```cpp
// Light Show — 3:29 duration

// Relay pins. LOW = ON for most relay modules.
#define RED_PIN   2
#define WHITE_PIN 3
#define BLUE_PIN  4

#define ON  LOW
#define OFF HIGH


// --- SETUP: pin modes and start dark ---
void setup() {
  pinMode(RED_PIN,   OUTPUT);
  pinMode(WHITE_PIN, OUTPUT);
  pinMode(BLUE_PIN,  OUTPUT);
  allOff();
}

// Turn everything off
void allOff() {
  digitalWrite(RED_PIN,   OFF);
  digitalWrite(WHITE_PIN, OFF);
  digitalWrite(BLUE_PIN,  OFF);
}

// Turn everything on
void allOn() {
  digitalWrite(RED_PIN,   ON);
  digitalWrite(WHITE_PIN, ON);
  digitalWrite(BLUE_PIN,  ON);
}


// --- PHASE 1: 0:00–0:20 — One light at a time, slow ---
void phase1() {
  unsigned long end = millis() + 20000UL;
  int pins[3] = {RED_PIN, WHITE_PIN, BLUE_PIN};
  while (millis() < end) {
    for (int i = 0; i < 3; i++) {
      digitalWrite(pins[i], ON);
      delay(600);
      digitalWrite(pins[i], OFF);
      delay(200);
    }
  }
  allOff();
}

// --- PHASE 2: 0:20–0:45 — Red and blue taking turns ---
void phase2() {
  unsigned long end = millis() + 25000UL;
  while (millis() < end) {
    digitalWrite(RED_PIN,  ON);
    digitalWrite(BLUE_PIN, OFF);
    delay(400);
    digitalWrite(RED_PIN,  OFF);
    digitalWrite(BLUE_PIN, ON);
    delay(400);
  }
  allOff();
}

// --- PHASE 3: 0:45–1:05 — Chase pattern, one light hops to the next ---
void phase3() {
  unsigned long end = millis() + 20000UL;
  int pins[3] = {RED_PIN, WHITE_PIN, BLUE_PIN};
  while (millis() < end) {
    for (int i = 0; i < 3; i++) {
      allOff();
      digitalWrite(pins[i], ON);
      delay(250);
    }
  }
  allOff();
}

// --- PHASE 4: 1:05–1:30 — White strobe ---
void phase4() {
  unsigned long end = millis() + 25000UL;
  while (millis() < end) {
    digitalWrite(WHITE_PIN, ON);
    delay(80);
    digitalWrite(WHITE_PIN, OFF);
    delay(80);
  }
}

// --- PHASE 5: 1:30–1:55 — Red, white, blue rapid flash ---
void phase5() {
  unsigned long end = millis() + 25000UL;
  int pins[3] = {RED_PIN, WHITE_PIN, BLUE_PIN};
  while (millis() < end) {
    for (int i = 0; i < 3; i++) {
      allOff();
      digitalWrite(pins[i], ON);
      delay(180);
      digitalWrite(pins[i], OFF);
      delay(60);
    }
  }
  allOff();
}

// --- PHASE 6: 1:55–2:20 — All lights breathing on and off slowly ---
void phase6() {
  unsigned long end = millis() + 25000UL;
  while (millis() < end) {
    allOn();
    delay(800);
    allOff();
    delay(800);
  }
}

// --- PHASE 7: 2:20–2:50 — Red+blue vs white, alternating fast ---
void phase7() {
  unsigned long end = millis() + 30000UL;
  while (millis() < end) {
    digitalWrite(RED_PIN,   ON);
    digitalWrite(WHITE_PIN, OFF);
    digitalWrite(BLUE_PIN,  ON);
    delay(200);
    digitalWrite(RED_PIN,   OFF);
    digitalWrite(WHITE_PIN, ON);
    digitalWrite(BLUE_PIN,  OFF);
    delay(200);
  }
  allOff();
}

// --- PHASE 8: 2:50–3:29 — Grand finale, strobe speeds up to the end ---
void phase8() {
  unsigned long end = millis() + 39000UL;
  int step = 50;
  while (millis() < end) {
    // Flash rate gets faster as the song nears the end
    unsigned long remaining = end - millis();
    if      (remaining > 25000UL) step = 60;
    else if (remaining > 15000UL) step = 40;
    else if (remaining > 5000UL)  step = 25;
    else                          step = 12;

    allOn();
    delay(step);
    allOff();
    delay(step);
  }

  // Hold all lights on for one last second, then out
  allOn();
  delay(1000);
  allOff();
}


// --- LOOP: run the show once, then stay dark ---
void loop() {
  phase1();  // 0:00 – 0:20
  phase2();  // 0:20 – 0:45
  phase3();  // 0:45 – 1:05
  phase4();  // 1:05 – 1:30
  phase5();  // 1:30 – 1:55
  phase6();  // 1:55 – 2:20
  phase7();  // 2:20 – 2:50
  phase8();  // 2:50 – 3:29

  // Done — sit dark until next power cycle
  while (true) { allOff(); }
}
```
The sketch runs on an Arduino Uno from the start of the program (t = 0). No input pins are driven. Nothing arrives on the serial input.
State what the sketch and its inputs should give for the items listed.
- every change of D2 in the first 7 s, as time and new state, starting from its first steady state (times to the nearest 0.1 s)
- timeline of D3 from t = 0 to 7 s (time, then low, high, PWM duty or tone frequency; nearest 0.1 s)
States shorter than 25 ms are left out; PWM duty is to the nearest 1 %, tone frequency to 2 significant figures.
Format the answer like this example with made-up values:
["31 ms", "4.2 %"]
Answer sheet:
["0 s low; 0.6 s high; 2.4 s low; 3 s high; 4.8 s low; 5.4 s high", "0 s high; 0.8 s low; 1.4 s high; 3.2 s low; 3.8 s high; 5.6 s low; 6.2 s high"]
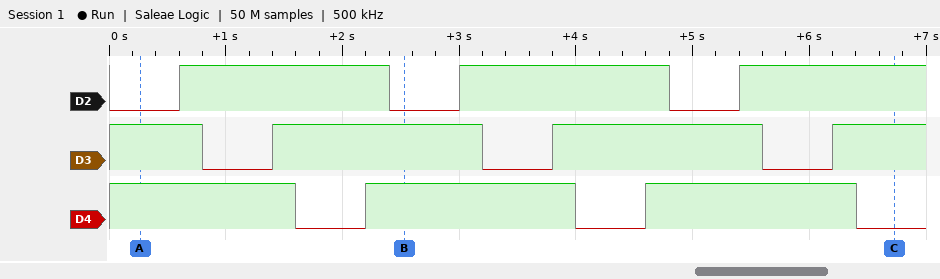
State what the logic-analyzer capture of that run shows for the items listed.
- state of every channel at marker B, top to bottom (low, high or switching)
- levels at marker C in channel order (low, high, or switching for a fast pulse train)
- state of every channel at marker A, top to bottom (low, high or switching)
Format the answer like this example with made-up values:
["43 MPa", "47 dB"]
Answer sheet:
["D2 low, D3 high, D4 high", "D2 high, D3 high, D4 low", "D2 low, D3 high, D4 high"]
